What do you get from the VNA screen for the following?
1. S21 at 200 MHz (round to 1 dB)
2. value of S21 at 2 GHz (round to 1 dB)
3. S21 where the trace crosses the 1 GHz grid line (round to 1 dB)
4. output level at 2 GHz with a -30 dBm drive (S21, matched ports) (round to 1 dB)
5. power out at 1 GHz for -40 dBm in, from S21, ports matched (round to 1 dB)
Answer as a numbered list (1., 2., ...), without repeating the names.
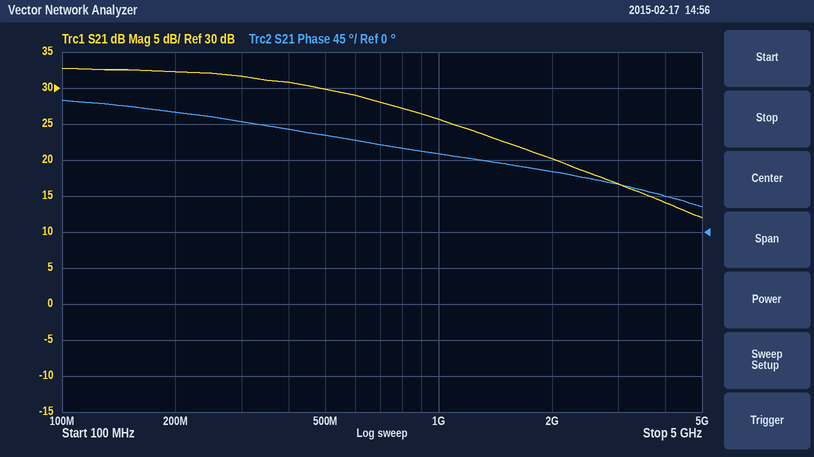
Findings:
1. 32 dB
2. 20 dB
3. 26 dB
4. -10 dBm
5. -14 dBm
